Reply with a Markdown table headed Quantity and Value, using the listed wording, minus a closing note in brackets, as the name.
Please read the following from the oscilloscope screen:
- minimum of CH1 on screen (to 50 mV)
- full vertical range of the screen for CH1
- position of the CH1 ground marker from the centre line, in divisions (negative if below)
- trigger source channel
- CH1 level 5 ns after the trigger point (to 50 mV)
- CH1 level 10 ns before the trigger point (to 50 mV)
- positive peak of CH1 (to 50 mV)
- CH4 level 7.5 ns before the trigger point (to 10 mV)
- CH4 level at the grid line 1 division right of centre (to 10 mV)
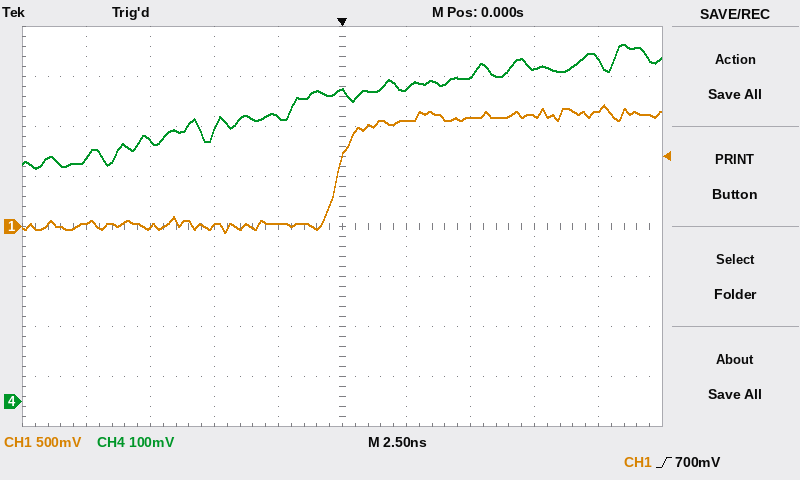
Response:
| Quantity | Value |
|---|---|
| minimum of CH1 on screen | -50 mV |
| full vertical range of the screen for CH1 | 4 V |
| position of the CH1 ground marker from the centre line, in divisions | 0.0 div |
| trigger source channel | CH1 |
| CH1 level 5 ns after the trigger point | 1.10 V |
| CH1 level 10 ns before the trigger point | 50 mV |
| positive peak of CH1 | 1.20 V |
| CH4 level 7.5 ns before the trigger point | 520 mV |
| CH4 level at the grid line 1 division right of centre | 630 mV |
